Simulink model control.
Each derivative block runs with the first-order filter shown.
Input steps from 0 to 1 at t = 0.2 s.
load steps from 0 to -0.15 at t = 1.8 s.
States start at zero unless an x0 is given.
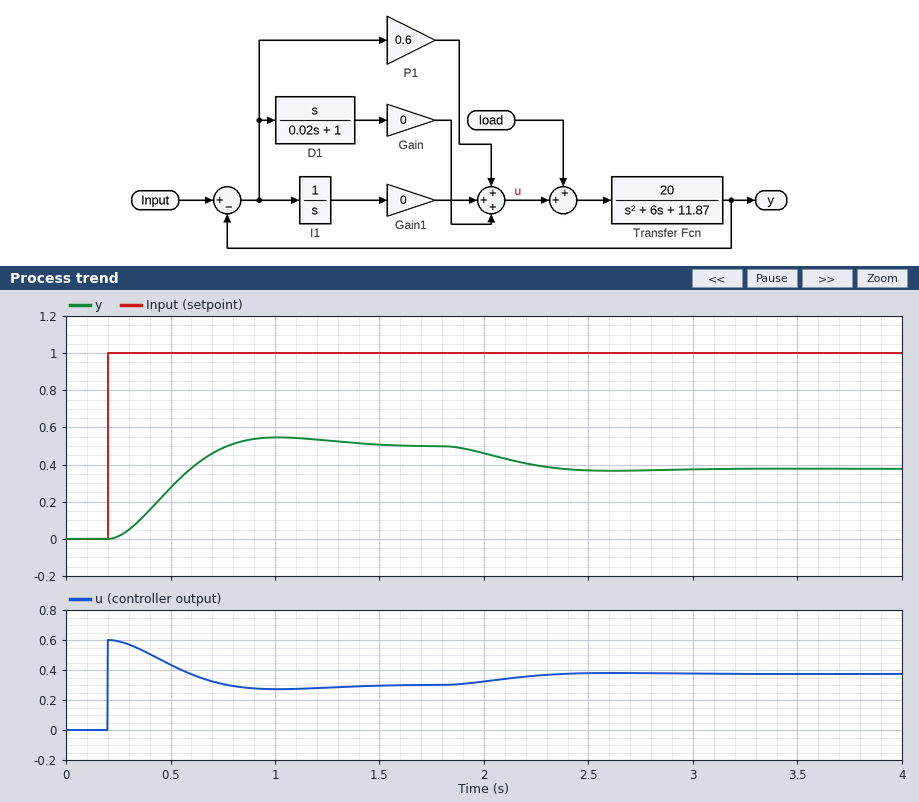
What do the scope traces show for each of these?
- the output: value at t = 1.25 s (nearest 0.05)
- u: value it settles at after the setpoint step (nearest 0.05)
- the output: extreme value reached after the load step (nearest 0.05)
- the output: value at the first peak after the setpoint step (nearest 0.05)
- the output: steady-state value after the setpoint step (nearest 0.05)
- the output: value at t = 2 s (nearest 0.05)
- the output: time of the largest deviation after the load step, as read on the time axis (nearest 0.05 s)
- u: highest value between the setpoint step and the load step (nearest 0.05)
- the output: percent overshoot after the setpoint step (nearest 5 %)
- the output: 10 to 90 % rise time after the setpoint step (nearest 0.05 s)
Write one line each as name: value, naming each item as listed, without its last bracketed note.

the output: value at t = 1.25 s: 0.55
u: value it settles at after the setpoint step: 0.30
the output: extreme value reached after the load step: 0.35
the output: value at the first peak after the setpoint step: 0.55
the output: steady-state value after the setpoint step: 0.50
the output: value at t = 2 s: 0.45
the output: time of the largest deviation after the load step, as read on the time axis: 2.60 s
u: highest value between the setpoint step and the load step: 0.60
the output: percent overshoot after the setpoint step: 10 %
the output: 10 to 90 % rise time after the setpoint step: 0.40 s
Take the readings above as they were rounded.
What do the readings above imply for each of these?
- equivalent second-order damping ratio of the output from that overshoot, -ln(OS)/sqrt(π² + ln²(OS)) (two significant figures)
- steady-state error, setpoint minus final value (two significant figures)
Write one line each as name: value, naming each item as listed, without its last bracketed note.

equivalent second-order damping ratio of the output from that overshoot, -ln(OS)/sqrt(π² + ln²(OS)): 0.59
steady-state error, setpoint minus final value: 0.50
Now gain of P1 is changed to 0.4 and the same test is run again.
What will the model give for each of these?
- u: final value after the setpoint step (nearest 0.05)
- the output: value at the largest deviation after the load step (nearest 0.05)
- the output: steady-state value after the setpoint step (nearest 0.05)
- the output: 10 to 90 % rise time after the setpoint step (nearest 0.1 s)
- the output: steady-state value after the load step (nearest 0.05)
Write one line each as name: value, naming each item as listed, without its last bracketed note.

u: final value after the setpoint step: 0.25
the output: value at the largest deviation after the load step: 0.25
the output: steady-state value after the setpoint step: 0.40
the output: 10 to 90 % rise time after the setpoint step: 0.5 s
the output: steady-state value after the load step: 0.25
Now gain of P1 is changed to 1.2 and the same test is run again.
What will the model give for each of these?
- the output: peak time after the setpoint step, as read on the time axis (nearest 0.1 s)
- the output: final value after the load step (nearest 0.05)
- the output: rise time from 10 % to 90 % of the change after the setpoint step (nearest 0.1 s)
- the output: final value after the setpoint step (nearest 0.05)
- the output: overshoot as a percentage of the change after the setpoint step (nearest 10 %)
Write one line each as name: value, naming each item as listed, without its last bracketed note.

the output: peak time after the setpoint step, as read on the time axis: 0.8 s
the output: final value after the load step: 0.60
the output: rise time from 10 % to 90 % of the change after the setpoint step: 0.3 s
the output: final value after the setpoint step: 0.65
the output: overshoot as a percentage of the change after the setpoint step: 20 %
